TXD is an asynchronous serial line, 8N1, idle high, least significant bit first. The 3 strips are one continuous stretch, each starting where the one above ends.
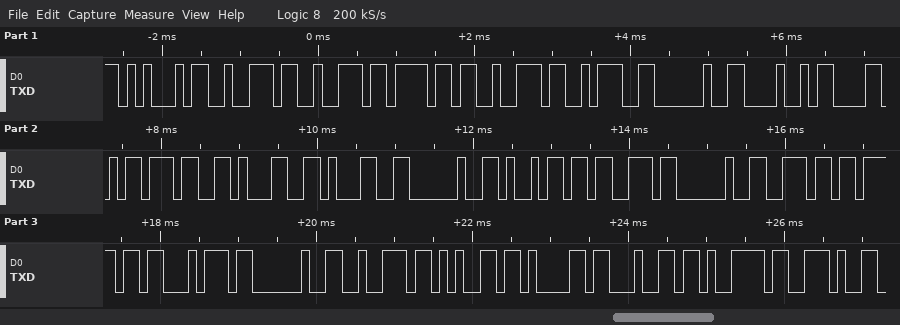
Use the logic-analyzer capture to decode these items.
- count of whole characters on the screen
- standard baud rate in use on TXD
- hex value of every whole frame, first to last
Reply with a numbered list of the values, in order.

1. 26
2. 9600 baud
3. 45 72 72 6F 72 3A 20 48 58 37 31 31 20 69 73 20 6E 6F 74 20 72 65 61 64 79 2E
